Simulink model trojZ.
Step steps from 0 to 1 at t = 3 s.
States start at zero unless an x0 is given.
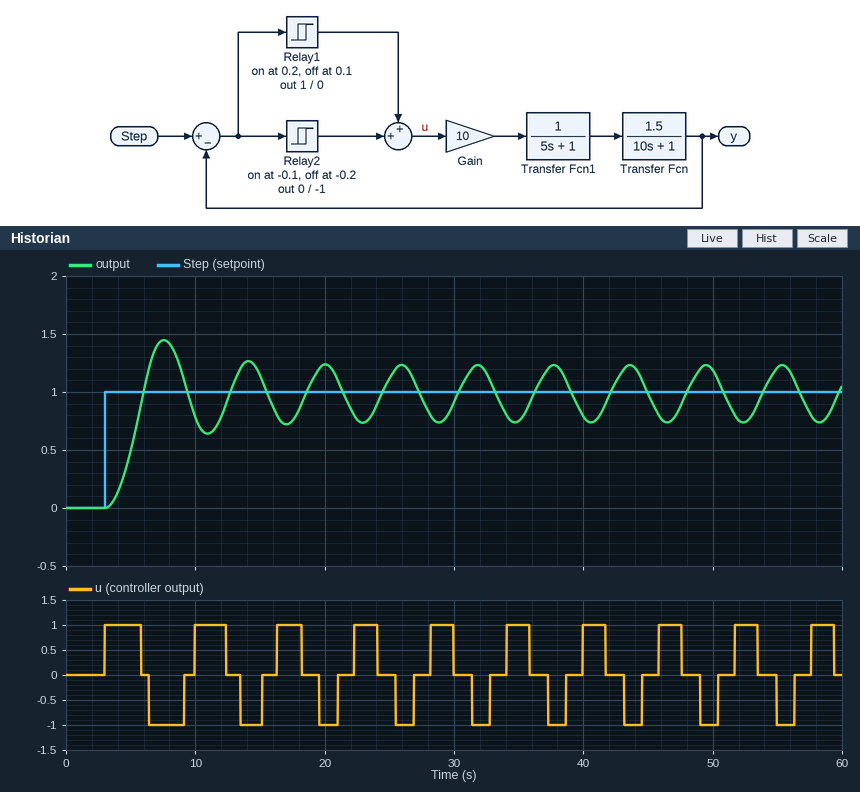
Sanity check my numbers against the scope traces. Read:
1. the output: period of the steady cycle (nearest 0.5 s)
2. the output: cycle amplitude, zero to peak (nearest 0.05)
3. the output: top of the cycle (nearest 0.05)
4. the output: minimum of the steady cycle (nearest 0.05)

6.0 s
0.25
1.25
0.75
